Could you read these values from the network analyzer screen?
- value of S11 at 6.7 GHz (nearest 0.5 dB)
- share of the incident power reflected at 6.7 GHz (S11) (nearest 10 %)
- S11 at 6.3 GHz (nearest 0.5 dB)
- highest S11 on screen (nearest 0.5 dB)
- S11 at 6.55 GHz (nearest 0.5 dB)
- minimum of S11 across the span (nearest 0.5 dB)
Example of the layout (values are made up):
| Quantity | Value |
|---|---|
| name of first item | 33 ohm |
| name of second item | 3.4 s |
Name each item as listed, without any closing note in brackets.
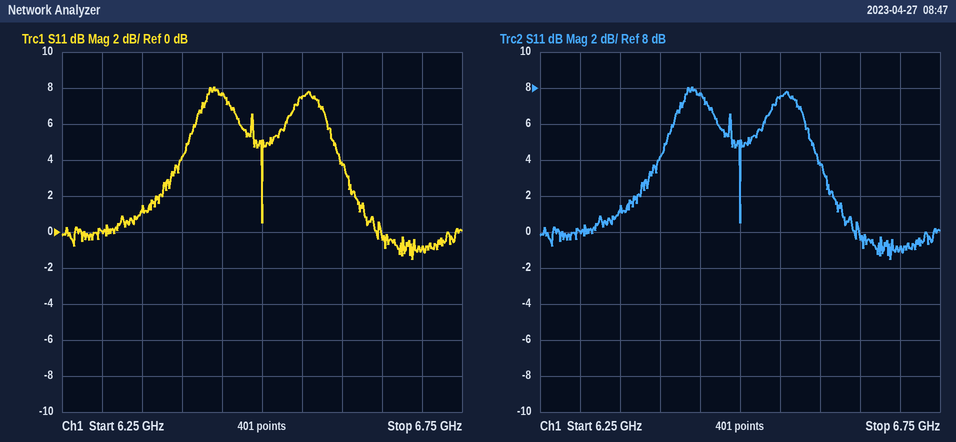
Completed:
| Quantity | Value |
|---|---|
| value of S11 at 6.7 GHz | -1.0 dB |
| share of the incident power reflected at 6.7 GHz (S11) | 80 % |
| S11 at 6.3 GHz | 0.0 dB |
| highest S11 on screen | 8.0 dB |
| S11 at 6.55 GHz | 7.5 dB |
| minimum of S11 across the span | -1.5 dB |
